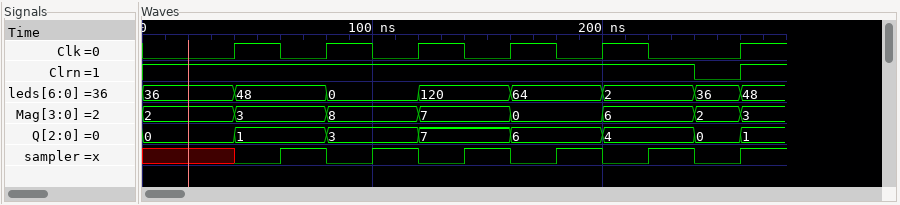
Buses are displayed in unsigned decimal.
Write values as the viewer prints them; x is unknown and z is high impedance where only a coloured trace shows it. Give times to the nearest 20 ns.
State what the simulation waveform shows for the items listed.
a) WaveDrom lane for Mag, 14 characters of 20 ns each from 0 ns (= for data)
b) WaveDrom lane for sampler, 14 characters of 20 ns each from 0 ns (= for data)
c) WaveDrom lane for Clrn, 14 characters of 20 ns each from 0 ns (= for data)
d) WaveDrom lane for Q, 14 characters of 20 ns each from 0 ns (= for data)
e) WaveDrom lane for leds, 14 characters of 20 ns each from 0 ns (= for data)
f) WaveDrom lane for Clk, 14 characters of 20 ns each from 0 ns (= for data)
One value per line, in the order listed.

{name: 'Mag', wave: '=.=.=.=.=.=.==', data: '2 3 8 7 0 6 2 3'}
{name: 'sampler', wave: 'x.010101010101'}
{name: 'Clrn', wave: '1...........01'}
{name: 'Q', wave: '=.=.=.=.=.=.==', data: '0 1 3 7 6 4 0 1'}
{name: 'leds', wave: '=.=.=.=.=.=.==', data: '36 48 0 120 64 2 36 48'}
{name: 'Clk', wave: '0.1010101010.1'}
